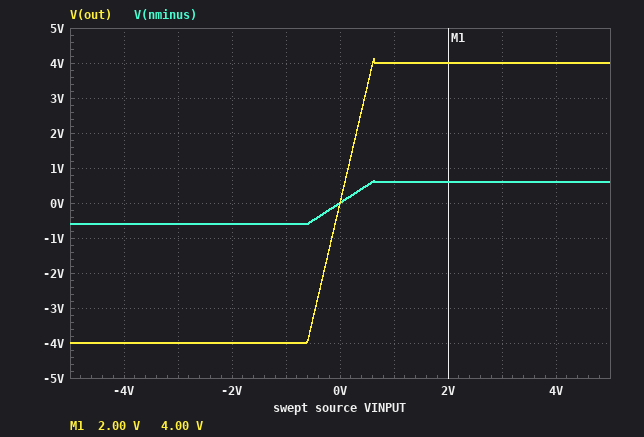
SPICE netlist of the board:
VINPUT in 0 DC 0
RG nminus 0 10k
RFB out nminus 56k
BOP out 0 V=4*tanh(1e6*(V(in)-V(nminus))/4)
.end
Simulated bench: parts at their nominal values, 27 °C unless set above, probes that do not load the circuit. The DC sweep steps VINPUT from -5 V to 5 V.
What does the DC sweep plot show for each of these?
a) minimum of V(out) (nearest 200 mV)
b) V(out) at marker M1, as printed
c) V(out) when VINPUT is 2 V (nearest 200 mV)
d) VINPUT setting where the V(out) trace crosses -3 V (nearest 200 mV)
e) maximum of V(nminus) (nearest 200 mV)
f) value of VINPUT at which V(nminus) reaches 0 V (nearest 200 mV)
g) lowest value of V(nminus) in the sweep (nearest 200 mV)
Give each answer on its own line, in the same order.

-4.0 V
4.00 V
4.0 V
-400 mV
600 mV
0 V
-600 mV
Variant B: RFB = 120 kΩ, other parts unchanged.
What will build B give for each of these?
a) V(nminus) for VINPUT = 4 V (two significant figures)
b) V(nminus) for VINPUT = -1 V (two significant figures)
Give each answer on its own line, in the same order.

310 mV
-310 mV
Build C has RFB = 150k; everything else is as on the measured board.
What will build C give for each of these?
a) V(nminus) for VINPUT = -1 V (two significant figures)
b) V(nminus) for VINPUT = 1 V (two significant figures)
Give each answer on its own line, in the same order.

-250 mV
250 mV
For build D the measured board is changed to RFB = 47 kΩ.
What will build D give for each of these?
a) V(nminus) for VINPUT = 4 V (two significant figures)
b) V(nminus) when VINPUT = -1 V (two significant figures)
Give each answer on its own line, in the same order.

700 mV
-700 mV
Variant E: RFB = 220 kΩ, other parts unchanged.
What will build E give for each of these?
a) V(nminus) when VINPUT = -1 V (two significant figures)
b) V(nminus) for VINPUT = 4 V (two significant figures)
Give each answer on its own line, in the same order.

-170 mV
170 mV
